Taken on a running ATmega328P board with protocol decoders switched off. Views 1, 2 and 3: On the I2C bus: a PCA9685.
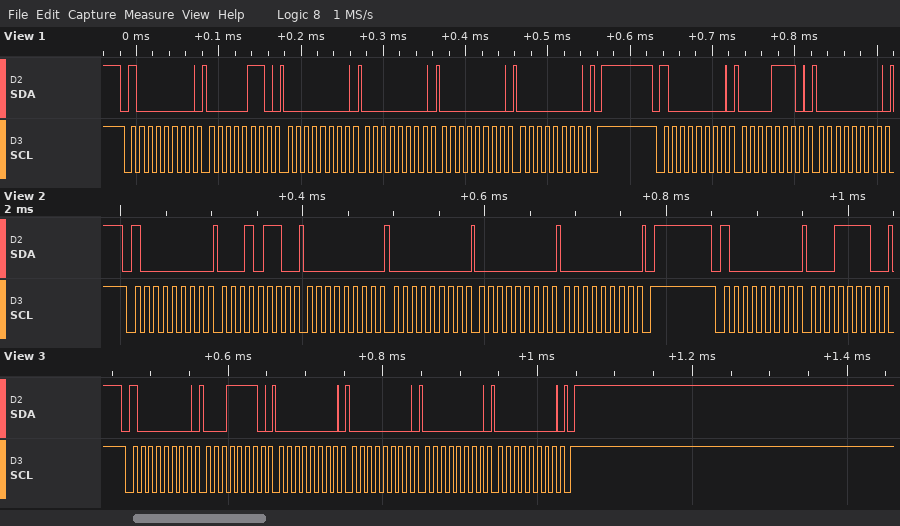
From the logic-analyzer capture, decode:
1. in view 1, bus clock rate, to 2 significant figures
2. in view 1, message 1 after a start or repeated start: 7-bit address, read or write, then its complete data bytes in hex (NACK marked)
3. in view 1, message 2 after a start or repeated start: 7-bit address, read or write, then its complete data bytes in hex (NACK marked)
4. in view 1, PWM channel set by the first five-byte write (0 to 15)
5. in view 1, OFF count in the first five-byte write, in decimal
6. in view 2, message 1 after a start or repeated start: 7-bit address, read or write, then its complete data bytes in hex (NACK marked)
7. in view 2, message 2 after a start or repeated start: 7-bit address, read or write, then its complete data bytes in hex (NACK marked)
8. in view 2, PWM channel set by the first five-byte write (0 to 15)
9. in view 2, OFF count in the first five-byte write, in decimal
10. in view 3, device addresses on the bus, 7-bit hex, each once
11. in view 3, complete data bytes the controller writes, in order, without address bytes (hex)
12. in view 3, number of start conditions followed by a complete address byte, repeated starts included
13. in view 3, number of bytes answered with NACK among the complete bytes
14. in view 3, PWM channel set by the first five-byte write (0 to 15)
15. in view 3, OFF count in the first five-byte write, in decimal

100 kHz
0x40 write: 06 00 00 00 00
0x40 write: 0E 00
0
0
0x40 write: 16 00 00 00 00
0x40 write: 1E
4
0
0x40
1E 00 00 00 00
1
0
6
0
